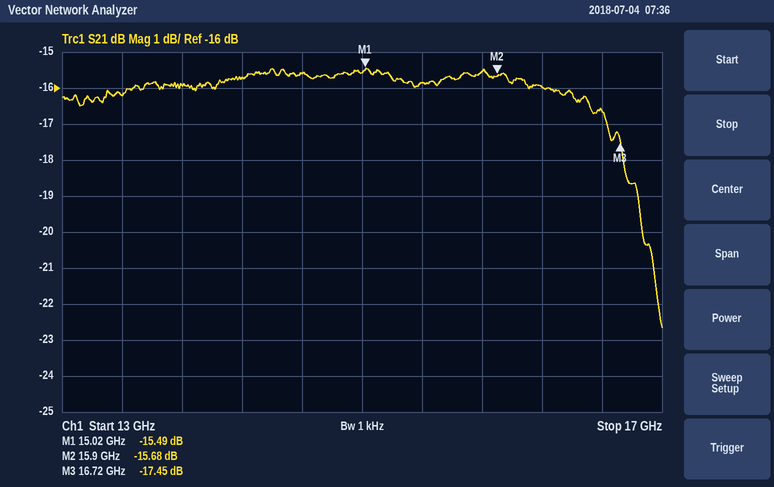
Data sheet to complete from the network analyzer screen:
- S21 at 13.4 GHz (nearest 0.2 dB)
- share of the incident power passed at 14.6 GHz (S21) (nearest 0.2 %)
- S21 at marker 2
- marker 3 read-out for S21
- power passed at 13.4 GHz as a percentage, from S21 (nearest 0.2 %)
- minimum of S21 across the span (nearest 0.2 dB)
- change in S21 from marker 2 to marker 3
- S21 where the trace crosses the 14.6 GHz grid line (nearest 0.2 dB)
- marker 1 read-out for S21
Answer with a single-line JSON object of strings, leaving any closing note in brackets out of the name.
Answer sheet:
{"S21 at 13.4 GHz": "-16.2 dB", "share of the incident power passed at 14.6 GHz (S21)": "2.8 %", "S21 at marker 2": "-15.68 dB", "marker 3 read-out for S21": "-17.45 dB", "power passed at 13.4 GHz as a percentage, from S21": "2.4 %", "minimum of S21 across the span": "-22.6 dB", "change in S21 from marker 2 to marker 3": "-1.77 dB", "S21 where the trace crosses the 14.6 GHz grid line": "-15.6 dB", "marker 1 read-out for S21": "-15.49 dB"}
